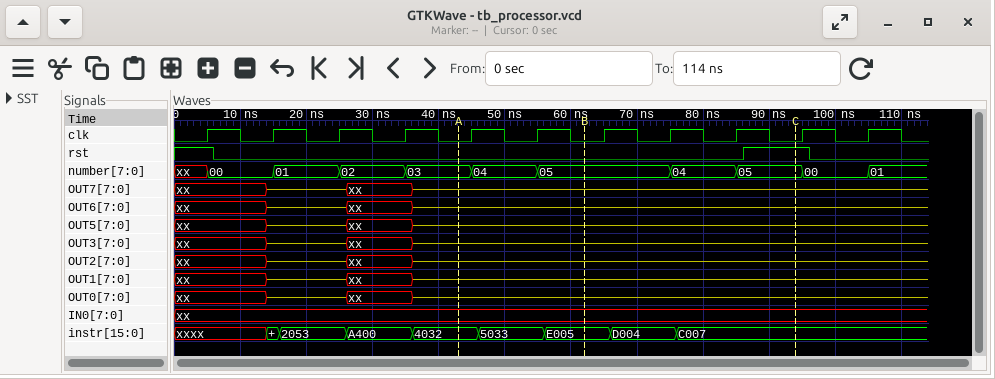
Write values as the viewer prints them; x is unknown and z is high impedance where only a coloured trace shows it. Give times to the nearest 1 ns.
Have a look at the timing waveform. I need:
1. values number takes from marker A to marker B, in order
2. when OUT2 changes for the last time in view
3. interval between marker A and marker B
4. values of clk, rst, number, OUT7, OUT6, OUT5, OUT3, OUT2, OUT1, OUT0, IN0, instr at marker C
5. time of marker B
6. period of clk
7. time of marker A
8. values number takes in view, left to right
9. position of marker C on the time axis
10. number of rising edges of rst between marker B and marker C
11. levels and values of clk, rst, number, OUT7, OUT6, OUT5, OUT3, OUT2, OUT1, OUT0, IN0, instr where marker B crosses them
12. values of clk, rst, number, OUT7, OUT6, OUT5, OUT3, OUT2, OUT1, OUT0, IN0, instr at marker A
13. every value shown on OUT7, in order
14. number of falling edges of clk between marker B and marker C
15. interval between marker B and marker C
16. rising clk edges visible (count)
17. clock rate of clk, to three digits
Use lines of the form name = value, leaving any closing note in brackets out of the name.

values number takes from marker A to marker B, in order = 03, 04, 05
when OUT2 changes for the last time in view = 36 ns
interval between marker A and marker B = 19 ns
values of clk, rst, number, OUT7, OUT6, OUT5, OUT3, OUT2, OUT1, OUT0, IN0, instr at marker C = clk=0, rst=1, number=05, OUT7=z, OUT6=z, OUT5=z, OUT3=z, OUT2=z, OUT1=z, OUT0=z, IN0=xx, instr=C007
time of marker B = 62 ns
period of clk = 10 ns
time of marker A = 43 ns
values number takes in view, left to right = xx, 00, 01, 02, 03, 04, 05, 04, 05, 00, 01
position of marker C on the time axis = 94 ns
number of rising edges of rst between marker B and marker C = 1
levels and values of clk, rst, number, OUT7, OUT6, OUT5, OUT3, OUT2, OUT1, OUT0, IN0, instr where marker B crosses them = clk=0, rst=0, number=05, OUT7=z, OUT6=z, OUT5=z, OUT3=z, OUT2=z, OUT1=z, OUT0=z, IN0=xx, instr=E005
values of clk, rst, number, OUT7, OUT6, OUT5, OUT3, OUT2, OUT1, OUT0, IN0, instr at marker A = clk=0, rst=0, number=03, OUT7=z, OUT6=z, OUT5=z, OUT3=z, OUT2=z, OUT1=z, OUT0=z, IN0=xx, instr=4032
every value shown on OUT7, in order = xx, z, xx, z
number of falling edges of clk between marker B and marker C = 3
interval between marker B and marker C = 32 ns
rising clk edges visible = 11
clock rate of clk, to three digits = 100 MHz
